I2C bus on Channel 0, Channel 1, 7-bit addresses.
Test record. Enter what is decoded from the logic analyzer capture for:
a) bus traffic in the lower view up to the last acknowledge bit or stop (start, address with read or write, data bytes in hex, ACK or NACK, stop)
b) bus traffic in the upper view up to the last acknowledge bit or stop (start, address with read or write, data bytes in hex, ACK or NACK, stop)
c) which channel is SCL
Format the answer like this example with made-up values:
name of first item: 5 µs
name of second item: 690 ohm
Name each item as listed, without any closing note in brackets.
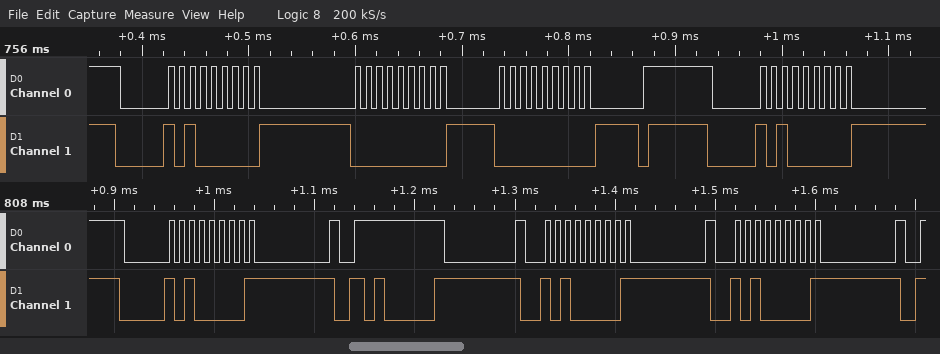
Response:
bus traffic in the lower view up to the last acknowledge bit or stop: start, address 50 write NACK, repeated start, address 74 write ACK, repeated start, address 50 write NACK
bus traffic in the upper view up to the last acknowledge bit or stop: start, address 50 write ACK, 00 ACK, 00 ACK, stop, start, address 50 write ACK
which channel is SCL: Channel 0
